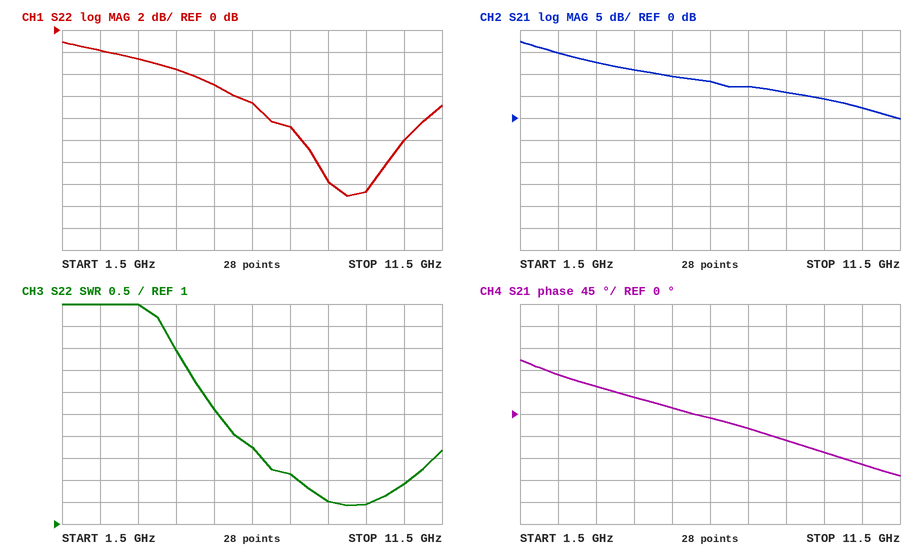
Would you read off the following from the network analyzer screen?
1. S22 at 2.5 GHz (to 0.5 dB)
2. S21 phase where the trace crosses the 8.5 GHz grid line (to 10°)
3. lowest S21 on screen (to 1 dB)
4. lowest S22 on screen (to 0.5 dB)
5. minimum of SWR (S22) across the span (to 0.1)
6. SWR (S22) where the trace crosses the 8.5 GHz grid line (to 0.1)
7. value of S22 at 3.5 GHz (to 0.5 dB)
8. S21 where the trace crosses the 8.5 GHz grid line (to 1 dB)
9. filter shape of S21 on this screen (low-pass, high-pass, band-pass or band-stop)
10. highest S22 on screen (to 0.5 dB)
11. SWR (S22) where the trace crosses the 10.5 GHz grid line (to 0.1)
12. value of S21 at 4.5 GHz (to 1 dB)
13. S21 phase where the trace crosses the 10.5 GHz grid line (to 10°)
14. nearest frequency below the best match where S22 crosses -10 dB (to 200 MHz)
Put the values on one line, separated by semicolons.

-2.0 dB; -50°; 0 dB; -15.0 dB; 1.4; 1.5; -2.5 dB; 6 dB; low-pass; -1.0 dB; 1.9; 11 dB; -100°; 7.8 GHz
